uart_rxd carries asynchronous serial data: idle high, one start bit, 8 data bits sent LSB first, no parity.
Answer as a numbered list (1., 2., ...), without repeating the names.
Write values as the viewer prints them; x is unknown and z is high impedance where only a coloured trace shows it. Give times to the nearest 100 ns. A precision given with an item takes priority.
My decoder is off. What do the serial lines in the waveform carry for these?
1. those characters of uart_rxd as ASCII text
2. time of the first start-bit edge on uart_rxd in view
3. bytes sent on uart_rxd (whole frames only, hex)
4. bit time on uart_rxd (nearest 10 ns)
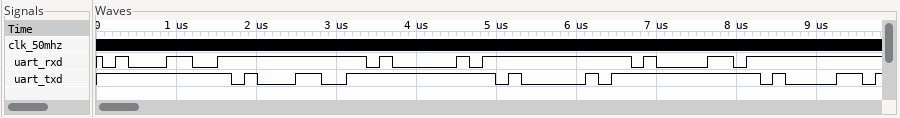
1. "1Aa"
2. 100 ns
3. 31, 41, 61
4. 160 ns
